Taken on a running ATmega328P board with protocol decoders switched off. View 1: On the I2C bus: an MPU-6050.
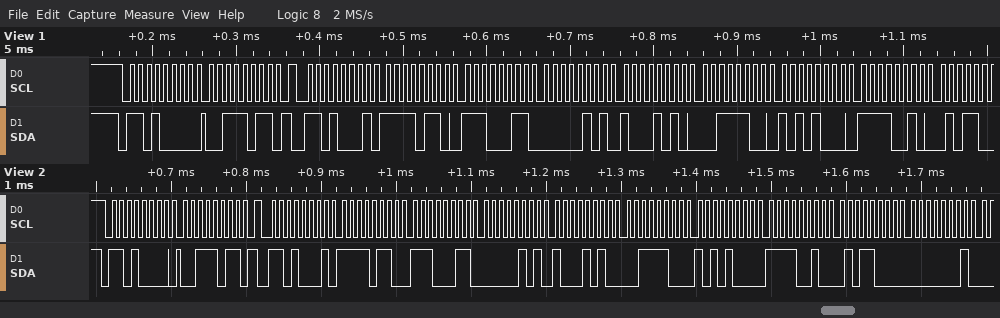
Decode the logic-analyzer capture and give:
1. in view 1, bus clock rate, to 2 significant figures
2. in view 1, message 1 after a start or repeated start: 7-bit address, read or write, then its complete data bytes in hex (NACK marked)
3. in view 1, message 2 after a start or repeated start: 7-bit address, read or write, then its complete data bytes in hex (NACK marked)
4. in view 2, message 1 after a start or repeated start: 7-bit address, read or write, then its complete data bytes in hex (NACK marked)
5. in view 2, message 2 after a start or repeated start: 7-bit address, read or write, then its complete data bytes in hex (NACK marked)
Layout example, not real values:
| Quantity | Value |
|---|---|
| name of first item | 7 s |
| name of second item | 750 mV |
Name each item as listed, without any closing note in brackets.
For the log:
| Quantity | Value |
|---|---|
| in view 1, bus clock rate, to 2 significant figures | 100 kHz |
| in view 1, message 1 after a start or repeated start: 7-bit address, read or write, then its complete data bytes in hex | 0x68 write: 3B |
| in view 1, message 2 after a start or repeated start: 7-bit address, read or write, then its complete data bytes in hex | 0x68 read: F6 E3 05 8A 3C A8 F2 |
| in view 2, message 1 after a start or repeated start: 7-bit address, read or write, then its complete data bytes in hex | 0x68 write: 3B |
| in view 2, message 2 after a start or repeated start: 7-bit address, read or write, then its complete data bytes in hex | 0x68 read: F6 E3 05 8A 3C A8 F2 58 01 |
